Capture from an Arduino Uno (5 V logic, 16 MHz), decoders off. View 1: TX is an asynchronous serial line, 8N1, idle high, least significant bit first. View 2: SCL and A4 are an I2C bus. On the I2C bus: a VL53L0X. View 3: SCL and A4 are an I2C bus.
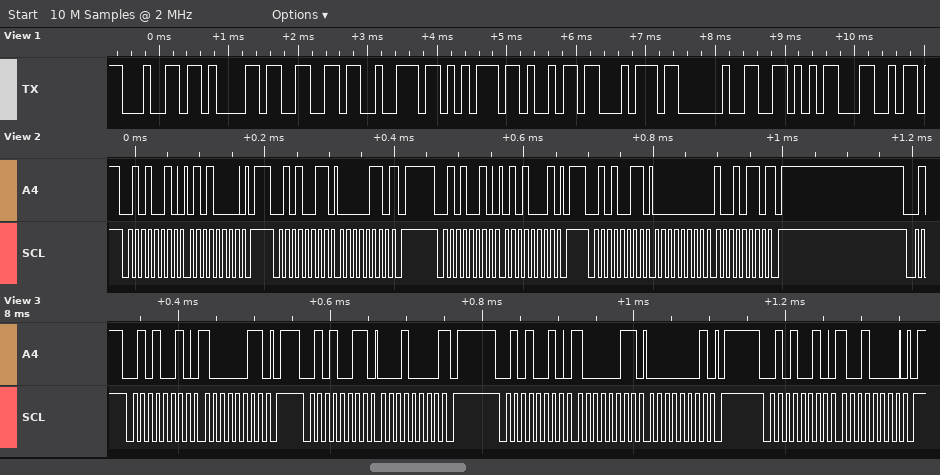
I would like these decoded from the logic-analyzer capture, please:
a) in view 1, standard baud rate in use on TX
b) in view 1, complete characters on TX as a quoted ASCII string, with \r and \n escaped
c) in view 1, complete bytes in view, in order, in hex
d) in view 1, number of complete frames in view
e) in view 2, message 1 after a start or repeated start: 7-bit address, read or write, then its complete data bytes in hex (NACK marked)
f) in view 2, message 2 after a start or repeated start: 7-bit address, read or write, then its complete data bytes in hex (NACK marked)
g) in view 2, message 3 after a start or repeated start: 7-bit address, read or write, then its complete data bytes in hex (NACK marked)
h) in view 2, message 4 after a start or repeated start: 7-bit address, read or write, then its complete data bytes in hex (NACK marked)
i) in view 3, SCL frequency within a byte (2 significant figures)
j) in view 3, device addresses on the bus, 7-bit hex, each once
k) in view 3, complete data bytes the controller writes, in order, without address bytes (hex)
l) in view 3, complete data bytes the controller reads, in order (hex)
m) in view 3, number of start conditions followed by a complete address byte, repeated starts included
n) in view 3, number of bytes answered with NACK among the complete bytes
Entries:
9600 baud
"dafruit VL"
64 61 66 72 75 69 74 20 56 4C
10
0x29 write: 50
0x29 read: 06 NACK
0x29 write: 51
0x29 read: 00 96 NACK
100 kHz
0x29
83 83 01 90
10
4
1
